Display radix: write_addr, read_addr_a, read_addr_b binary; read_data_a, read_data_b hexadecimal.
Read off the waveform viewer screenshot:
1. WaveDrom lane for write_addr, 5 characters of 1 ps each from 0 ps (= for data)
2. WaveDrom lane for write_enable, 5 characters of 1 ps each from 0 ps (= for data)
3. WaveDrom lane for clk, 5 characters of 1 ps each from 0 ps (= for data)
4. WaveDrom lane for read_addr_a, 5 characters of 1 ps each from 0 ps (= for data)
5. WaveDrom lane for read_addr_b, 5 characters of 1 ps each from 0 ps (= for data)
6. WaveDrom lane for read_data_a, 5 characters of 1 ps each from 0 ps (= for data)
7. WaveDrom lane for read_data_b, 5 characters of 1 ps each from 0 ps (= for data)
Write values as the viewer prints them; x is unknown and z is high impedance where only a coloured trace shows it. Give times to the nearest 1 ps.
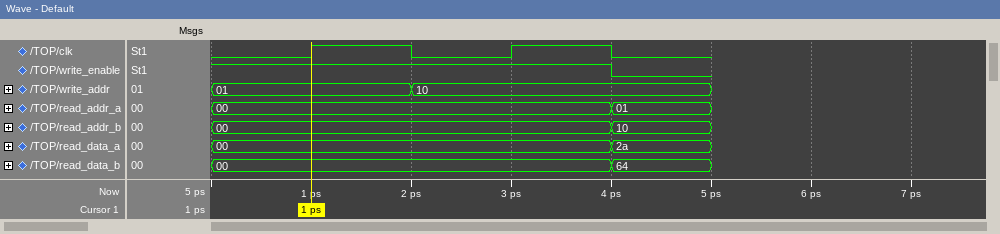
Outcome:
{name: 'write_addr', wave: '=.=..', data: '01 10'}
{name: 'write_enable', wave: '1...0'}
{name: 'clk', wave: '01010'}
{name: 'read_addr_a', wave: '=...=', data: '00 01'}
{name: 'read_addr_b', wave: '=...=', data: '00 10'}
{name: 'read_data_a', wave: '=...=', data: '00 2a'}
{name: 'read_data_b', wave: '=...=', data: '00 64'}
